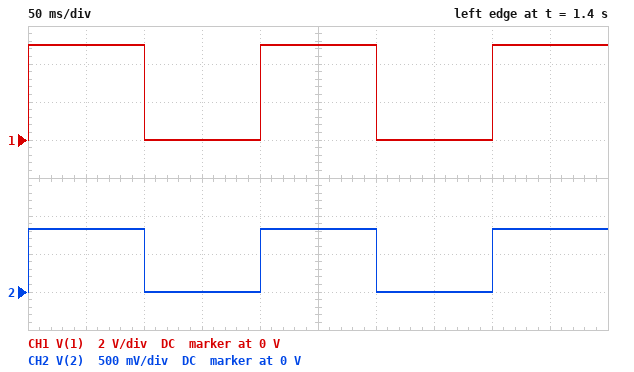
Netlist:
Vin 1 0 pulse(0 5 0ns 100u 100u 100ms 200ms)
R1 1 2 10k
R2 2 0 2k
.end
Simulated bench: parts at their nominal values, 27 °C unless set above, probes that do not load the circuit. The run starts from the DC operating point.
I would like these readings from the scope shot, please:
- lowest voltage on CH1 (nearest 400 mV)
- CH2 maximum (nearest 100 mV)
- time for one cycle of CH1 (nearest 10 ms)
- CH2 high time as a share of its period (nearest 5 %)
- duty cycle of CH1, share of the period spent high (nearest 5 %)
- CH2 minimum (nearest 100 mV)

0 V
800 mV
200 ms
50 %
50 %
0 V
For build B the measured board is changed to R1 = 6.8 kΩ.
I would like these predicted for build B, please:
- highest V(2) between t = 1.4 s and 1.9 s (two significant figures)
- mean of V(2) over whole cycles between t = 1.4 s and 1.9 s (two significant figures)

1.1 V
570 mV
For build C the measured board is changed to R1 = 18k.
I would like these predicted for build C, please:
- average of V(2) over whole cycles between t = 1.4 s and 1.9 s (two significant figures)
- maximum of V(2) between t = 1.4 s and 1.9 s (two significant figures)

250 mV
500 mV
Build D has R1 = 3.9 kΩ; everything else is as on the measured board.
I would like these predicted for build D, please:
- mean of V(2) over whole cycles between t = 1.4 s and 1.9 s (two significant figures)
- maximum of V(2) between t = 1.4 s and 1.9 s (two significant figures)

850 mV
1.7 V
